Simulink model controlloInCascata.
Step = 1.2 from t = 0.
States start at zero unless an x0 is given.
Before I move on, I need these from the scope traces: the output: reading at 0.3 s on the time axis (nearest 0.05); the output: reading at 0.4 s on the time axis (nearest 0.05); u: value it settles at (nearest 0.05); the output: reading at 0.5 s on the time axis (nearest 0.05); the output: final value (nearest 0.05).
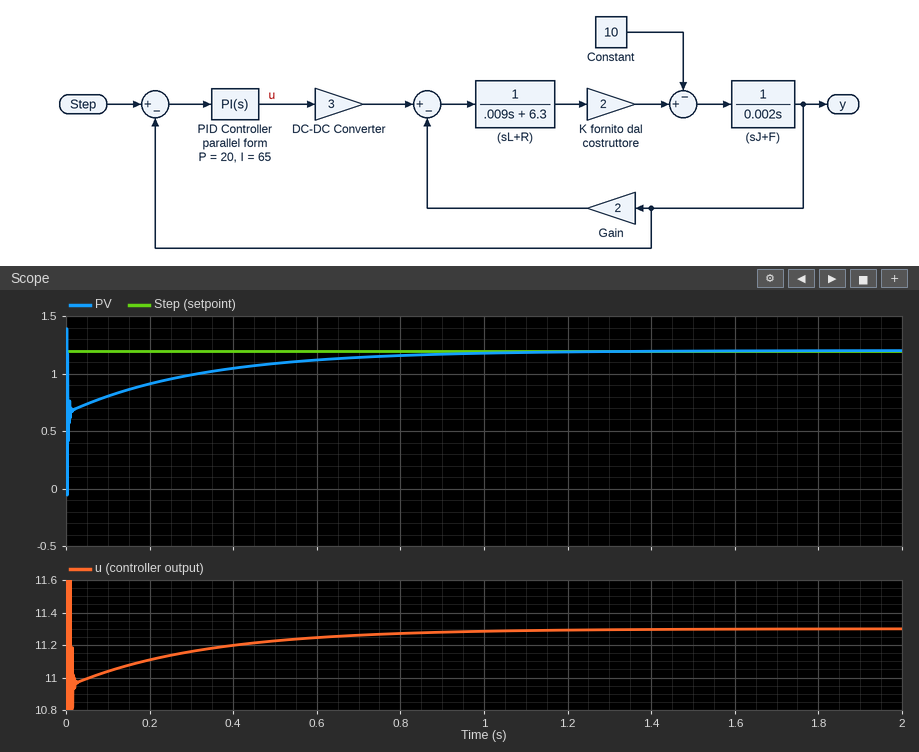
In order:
1.00
1.05
11.30
1.10
1.20
